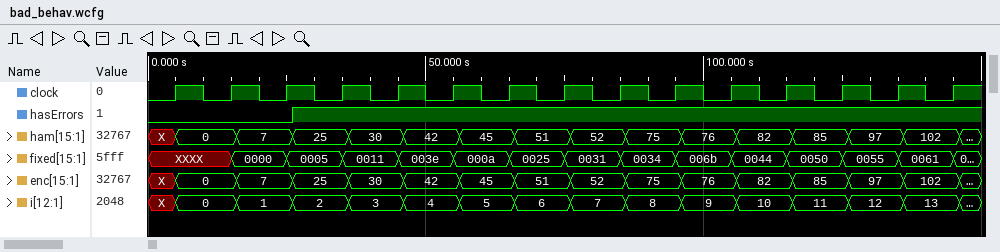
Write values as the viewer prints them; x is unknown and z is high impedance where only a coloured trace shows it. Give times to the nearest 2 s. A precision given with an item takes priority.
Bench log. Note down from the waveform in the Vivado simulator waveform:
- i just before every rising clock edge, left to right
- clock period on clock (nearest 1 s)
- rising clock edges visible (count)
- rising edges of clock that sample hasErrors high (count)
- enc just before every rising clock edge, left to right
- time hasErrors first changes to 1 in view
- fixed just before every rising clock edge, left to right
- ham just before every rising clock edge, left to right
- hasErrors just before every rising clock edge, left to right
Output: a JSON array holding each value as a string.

["X, 0, 1, 2, 3, 4, 5, 6, 7, 8, 9, 10, 11, 12, 13", "10 s", "15", "12", "X, 0, 7, 25, 30, 42, 45, 51, 52, 75, 76, 82, 85, 97, 102", "26 s", "XXXX, XXXX, 0000, 0005, 0011, 003e, 000a, 0025, 0031, 0034, 006b, 0044, 0050, 0055, 0061", "X, 0, 7, 25, 30, 42, 45, 51, 52, 75, 76, 82, 85, 97, 102", "0 0 0 1 1 1 1 1 1 1 1 1 1 1 1"]
